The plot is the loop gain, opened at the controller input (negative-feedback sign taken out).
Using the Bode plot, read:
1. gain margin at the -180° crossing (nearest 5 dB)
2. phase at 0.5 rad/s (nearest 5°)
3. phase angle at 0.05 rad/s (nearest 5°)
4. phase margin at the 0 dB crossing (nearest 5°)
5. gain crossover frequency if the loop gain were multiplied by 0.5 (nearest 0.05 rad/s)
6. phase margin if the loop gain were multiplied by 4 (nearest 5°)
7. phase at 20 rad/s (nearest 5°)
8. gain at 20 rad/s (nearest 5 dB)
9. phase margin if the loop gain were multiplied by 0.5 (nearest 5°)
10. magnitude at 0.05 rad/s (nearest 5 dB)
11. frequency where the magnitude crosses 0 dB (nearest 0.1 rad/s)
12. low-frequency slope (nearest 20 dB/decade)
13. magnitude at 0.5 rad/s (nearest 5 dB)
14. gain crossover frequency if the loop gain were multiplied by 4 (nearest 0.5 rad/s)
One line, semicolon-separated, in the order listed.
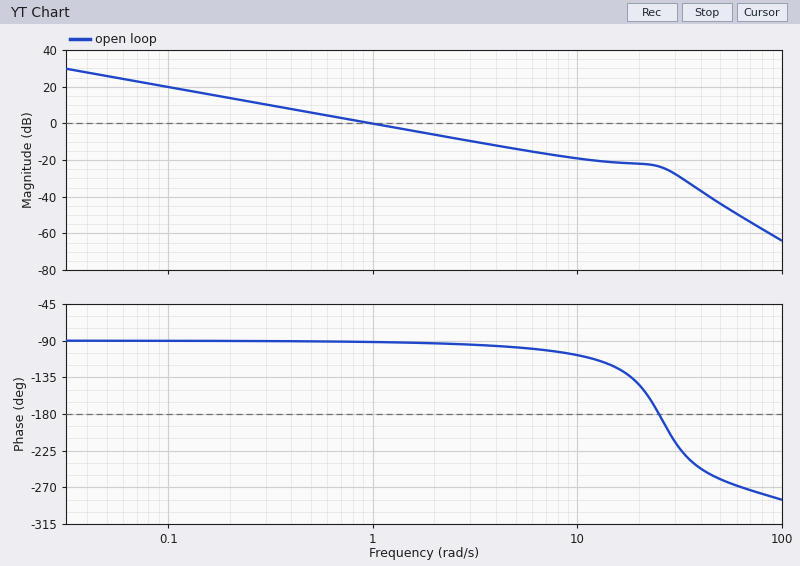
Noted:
25 dB; -90°; -90°; 90°; 0.50 rad/s; 85°; -145°; -20 dB; 90°; 25 dB; 1.0 rad/s; -20 dB/decade; 5 dB; 4.0 rad/s
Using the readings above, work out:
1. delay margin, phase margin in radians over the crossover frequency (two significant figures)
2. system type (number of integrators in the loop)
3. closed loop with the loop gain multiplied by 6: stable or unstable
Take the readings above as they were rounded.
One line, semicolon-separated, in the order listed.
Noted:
1.6 s; 1; stable
